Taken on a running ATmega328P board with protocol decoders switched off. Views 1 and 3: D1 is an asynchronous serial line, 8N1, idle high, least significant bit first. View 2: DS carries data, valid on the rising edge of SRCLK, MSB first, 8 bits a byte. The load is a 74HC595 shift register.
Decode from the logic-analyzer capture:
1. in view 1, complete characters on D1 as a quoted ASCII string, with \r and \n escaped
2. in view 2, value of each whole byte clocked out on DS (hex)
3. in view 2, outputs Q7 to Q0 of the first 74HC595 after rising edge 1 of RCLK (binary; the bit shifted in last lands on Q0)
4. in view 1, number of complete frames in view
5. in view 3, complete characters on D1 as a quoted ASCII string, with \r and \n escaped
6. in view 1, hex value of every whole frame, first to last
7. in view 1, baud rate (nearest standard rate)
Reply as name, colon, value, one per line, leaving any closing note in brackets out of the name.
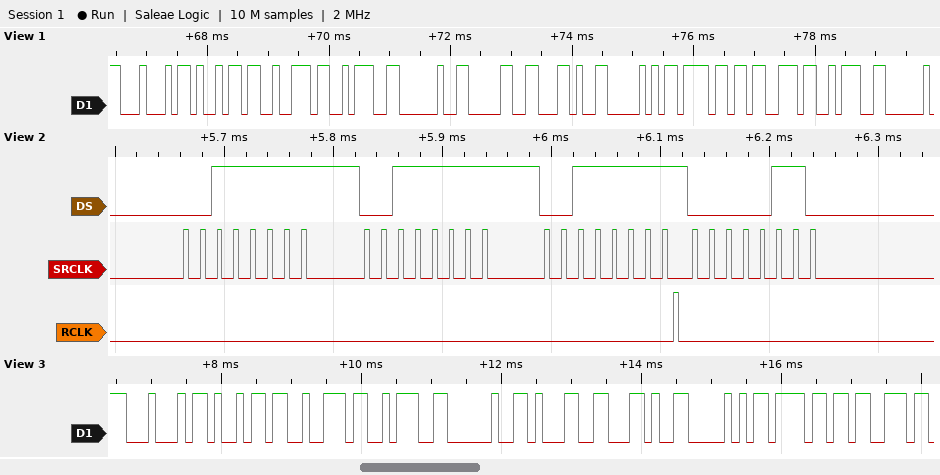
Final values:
in view 1, complete characters on D1 as a quoted ASCII string, with \r and \n escaped: "Dir: 0,Pos:"
in view 2, value of each whole byte clocked out on DS: 3F 3F 3F 06
in view 2, outputs Q7 to Q0 of the first 74HC595 after rising edge 1 of RCLK: 00111111
in view 1, number of complete frames in view: 11
in view 3, complete characters on D1 as a quoted ASCII string, with \r and \n escaped: "Dir: 1,Pos"
in view 1, hex value of every whole frame, first to last: 44 69 72 3A 20 30 2C 50 6F 73 3A
in view 1, baud rate: 9600 baud
